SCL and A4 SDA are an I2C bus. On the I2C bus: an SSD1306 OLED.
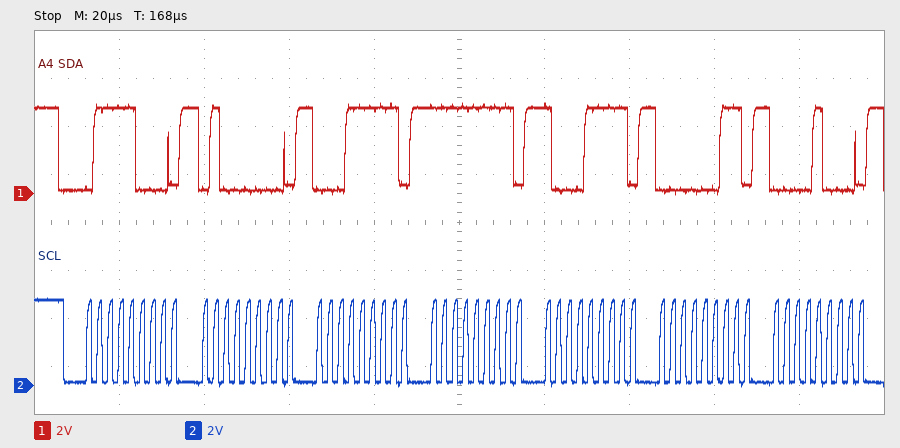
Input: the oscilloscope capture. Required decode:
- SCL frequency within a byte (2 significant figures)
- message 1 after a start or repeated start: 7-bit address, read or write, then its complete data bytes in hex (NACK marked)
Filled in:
400 kHz
0x3C write: 40 1F FF 8F 03 08
